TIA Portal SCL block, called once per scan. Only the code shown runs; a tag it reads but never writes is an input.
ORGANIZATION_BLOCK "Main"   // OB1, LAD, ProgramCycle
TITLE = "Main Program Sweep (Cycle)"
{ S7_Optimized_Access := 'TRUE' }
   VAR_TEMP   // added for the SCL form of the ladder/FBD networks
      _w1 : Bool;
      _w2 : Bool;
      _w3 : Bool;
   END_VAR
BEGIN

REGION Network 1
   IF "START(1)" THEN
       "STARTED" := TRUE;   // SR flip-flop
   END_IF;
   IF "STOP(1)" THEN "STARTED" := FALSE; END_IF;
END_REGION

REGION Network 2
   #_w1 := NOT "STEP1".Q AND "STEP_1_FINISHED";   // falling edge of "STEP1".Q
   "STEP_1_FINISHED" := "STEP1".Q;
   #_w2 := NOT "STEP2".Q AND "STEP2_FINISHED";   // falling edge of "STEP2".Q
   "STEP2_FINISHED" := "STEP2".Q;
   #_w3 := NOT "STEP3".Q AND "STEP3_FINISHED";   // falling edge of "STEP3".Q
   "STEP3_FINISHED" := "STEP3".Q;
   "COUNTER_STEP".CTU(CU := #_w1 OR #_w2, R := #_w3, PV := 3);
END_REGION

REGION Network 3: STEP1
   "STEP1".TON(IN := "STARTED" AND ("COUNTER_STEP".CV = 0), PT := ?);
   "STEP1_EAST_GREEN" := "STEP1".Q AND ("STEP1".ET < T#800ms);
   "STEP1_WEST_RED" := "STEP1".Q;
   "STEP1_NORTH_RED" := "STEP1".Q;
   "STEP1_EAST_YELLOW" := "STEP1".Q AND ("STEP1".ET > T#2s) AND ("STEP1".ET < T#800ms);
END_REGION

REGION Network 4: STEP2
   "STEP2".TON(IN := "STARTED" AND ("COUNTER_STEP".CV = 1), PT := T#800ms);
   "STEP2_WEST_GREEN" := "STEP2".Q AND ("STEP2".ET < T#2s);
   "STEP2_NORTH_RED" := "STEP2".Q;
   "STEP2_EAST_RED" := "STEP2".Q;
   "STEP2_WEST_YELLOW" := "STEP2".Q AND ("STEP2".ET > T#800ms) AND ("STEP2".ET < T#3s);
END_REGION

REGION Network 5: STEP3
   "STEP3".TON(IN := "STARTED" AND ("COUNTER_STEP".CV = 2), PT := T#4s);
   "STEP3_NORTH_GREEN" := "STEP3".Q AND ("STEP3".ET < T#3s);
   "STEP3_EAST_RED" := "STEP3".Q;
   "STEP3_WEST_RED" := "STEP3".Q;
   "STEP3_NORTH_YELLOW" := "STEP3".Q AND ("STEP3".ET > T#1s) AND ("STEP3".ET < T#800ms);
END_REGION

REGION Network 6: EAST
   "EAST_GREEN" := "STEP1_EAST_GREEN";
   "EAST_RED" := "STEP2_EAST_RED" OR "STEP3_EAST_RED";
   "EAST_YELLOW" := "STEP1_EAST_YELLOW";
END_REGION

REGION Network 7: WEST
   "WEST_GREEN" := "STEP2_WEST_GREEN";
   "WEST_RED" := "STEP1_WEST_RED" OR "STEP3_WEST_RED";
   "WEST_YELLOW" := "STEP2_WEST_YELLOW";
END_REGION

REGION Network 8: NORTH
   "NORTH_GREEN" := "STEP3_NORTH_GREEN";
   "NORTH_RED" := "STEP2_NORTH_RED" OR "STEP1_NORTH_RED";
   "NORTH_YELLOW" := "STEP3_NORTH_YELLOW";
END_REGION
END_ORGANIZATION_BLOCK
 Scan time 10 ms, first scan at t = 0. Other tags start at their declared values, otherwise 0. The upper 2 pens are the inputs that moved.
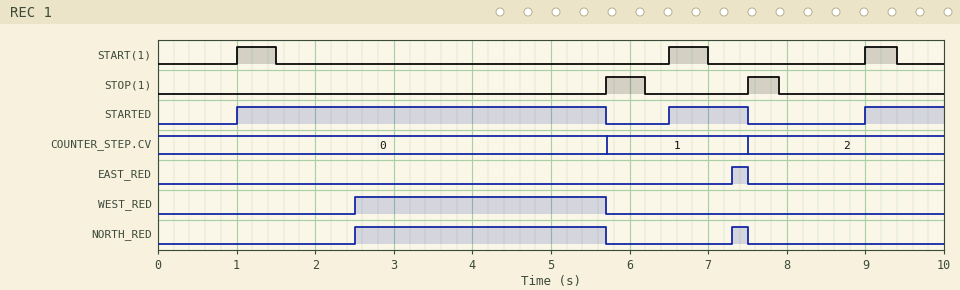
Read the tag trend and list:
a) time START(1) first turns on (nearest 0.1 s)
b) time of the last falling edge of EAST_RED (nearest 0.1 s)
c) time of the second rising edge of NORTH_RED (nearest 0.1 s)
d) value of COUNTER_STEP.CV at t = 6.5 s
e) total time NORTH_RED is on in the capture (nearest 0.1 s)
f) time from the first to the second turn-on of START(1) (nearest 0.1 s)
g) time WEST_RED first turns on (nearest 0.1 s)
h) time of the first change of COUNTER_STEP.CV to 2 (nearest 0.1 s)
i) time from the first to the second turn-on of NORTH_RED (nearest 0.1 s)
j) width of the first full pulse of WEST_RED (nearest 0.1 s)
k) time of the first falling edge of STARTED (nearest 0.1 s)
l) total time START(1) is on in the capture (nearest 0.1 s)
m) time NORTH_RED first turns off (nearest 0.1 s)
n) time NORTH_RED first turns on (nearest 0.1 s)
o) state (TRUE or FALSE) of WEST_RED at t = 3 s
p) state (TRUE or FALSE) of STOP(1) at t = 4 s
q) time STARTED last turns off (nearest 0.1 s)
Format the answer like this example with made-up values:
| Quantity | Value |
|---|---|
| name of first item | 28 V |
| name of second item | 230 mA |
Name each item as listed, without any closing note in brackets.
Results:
| Quantity | Value |
|---|---|
| time START(1) first turns on | 1.0 s |
| time of the last falling edge of EAST_RED | 7.5 s |
| time of the second rising edge of NORTH_RED | 7.3 s |
| value of COUNTER_STEP.CV at t = 6.5 s | 1 |
| total time NORTH_RED is on in the capture | 3.4 s |
| time from the first to the second turn-on of START(1) | 5.5 s |
| time WEST_RED first turns on | 2.5 s |
| time of the first change of COUNTER_STEP.CV to 2 | 7.5 s |
| time from the first to the second turn-on of NORTH_RED | 4.8 s |
| width of the first full pulse of WEST_RED | 3.2 s |
| time of the first falling edge of STARTED | 5.7 s |
| total time START(1) is on in the capture | 1.4 s |
| time NORTH_RED first turns off | 5.7 s |
| time NORTH_RED first turns on | 2.5 s |
| state (TRUE or FALSE) of WEST_RED at t = 3 s | TRUE |
| state (TRUE or FALSE) of STOP(1) at t = 4 s | FALSE |
| time STARTED last turns off | 7.5 s |
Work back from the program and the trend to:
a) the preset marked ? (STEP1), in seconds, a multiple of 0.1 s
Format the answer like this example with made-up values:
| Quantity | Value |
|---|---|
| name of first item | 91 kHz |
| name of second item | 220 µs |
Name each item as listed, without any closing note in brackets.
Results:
| Quantity | Value |
|---|---|
| the preset marked ? (STEP1), in seconds, a multiple of 0.1 s | 1.5 s |
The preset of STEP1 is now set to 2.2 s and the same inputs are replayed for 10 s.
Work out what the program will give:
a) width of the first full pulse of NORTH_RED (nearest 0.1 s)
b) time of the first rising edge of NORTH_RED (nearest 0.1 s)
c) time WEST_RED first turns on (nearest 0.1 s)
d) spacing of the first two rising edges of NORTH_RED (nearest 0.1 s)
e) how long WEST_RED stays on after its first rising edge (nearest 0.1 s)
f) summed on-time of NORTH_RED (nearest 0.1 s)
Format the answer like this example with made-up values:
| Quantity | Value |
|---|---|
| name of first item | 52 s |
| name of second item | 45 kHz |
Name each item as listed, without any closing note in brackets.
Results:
| Quantity | Value |
|---|---|
| width of the first full pulse of NORTH_RED | 2.5 s |
| time of the first rising edge of NORTH_RED | 3.2 s |
| time WEST_RED first turns on | 3.2 s |
| spacing of the first two rising edges of NORTH_RED | 4.1 s |
| how long WEST_RED stays on after its first rising edge | 2.5 s |
| summed on-time of NORTH_RED | 2.7 s |
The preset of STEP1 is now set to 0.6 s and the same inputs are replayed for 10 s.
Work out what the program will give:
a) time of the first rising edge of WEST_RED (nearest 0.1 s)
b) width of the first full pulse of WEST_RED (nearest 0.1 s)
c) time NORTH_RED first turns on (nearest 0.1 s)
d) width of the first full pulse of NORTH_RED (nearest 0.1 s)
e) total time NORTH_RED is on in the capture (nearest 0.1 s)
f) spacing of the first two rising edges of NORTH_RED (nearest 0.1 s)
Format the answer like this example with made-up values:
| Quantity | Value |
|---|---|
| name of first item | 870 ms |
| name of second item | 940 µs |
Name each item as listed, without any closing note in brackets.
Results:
| Quantity | Value |
|---|---|
| time of the first rising edge of WEST_RED | 1.6 s |
| width of the first full pulse of WEST_RED | 4.1 s |
| time NORTH_RED first turns on | 1.6 s |
| width of the first full pulse of NORTH_RED | 4.1 s |
| total time NORTH_RED is on in the capture | 4.3 s |
| spacing of the first two rising edges of NORTH_RED | 5.7 s |
